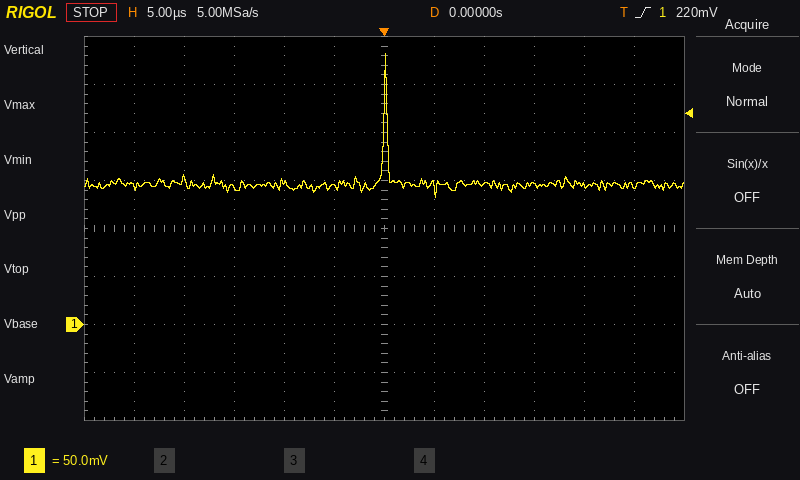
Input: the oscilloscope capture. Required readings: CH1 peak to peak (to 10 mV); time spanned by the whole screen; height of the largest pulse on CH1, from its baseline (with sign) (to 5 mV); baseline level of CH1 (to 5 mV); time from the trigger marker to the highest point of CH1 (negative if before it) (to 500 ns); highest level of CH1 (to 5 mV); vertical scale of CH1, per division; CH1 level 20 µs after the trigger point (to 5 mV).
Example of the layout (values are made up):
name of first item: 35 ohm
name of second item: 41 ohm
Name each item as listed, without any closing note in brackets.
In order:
CH1 peak to peak: 150 mV
time spanned by the whole screen: 60 µs
height of the largest pulse on CH1, from its baseline (with sign): +135 mV
baseline level of CH1: 145 mV
time from the trigger marker to the highest point of CH1 (negative if before it): 0.0 µs
highest level of CH1: 280 mV
vertical scale of CH1, per division: 50 mV
CH1 level 20 µs after the trigger point: 145 mV
